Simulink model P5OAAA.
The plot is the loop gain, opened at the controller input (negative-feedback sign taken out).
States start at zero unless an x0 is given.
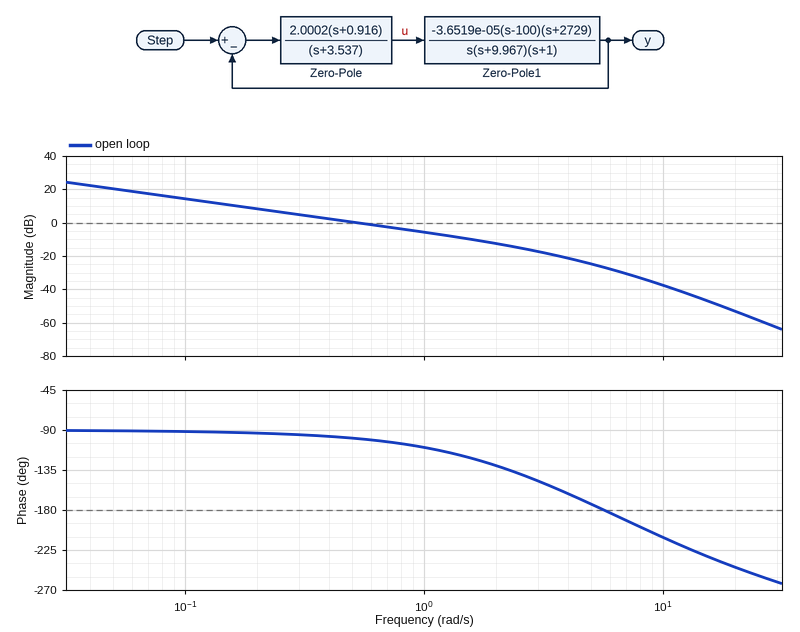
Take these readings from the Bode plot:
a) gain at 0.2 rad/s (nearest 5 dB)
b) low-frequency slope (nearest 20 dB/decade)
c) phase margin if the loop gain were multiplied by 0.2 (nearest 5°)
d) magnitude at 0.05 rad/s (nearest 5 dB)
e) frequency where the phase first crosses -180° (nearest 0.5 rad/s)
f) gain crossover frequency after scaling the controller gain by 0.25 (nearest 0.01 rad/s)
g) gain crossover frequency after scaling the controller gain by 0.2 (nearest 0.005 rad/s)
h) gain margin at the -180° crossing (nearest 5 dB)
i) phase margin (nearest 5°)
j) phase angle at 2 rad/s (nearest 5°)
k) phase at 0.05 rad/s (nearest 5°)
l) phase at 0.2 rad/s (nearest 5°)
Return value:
10 dB
-20 dB/decade
90°
20 dB
5.5 rad/s
0.13 rad/s
0.105 rad/s
25 dB
80°
-130°
-90°
-95°
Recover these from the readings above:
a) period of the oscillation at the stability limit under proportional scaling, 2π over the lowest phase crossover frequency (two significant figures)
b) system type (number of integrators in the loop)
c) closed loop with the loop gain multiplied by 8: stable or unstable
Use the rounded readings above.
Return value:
1.1 s
1
stable
